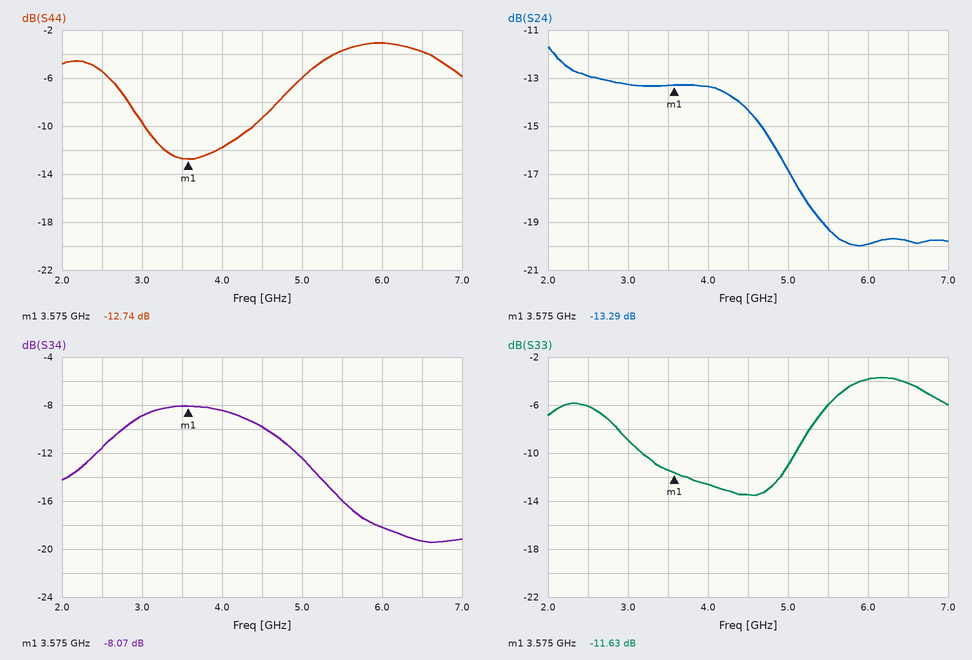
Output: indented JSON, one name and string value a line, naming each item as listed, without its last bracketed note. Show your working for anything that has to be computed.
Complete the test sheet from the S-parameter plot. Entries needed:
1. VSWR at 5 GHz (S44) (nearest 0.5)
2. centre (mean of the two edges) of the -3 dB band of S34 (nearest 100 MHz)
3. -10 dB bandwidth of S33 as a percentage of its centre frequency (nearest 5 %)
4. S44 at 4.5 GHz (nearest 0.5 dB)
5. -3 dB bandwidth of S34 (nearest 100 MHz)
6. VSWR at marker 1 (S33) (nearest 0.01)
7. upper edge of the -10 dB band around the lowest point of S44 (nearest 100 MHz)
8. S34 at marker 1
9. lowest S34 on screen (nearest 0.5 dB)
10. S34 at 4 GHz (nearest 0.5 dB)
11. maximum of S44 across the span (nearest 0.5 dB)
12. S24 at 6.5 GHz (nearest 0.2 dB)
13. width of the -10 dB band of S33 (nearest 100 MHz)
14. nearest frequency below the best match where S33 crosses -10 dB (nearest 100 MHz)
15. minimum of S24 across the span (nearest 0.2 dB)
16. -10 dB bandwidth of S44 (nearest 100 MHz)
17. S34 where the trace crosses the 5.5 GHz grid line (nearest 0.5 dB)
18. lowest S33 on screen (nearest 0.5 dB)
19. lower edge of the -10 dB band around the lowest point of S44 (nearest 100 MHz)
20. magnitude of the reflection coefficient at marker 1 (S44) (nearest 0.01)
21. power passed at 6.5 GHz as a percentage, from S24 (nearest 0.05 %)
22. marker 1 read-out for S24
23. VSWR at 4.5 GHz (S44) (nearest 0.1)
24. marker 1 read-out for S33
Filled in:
{
  "VSWR at 5 GHz (S44)": "|Γ| = 10^(-6/20) = 0.5012; VSWR = (1 + 0.5012)/(1 − 0.5012) ≈ 3.0",
  "centre (mean of the two edges) of the -3 dB band of S34": "3.7 GHz",
  "-10 dB bandwidth of S33 as a percentage of its centre frequency": "1.9 GHz / 4.15 GHz ≈ 45.8 %, so 45 % to the nearest 5 %",
  "S44 at 4.5 GHz": "-9.5 dB",
  "-3 dB bandwidth of S34": "4.8 GHz − 2.6 GHz = 2.2 GHz",
  "VSWR at marker 1 (S33)": "(1 + 0.2621)/(1 − 0.2621) ≈ 1.71",
  "upper edge of the -10 dB band around the lowest point of S44": "4.4 GHz",
  "S34 at marker 1": "-8.07 dB",
  "lowest S34 on screen": "-19.5 dB",
  "S34 at 4 GHz": "-8.5 dB",
  "maximum of S44 across the span": "-3.0 dB",
  "S24 at 6.5 GHz": "-19.8 dB",
  "width of the -10 dB band of S33": "5.1 GHz − 3.2 GHz = 1.9 GHz",
  "nearest frequency below the best match where S33 crosses -10 dB": "3.2 GHz",
  "minimum of S24 across the span": "-20.0 dB",
  "-10 dB bandwidth of S44": "4.4 GHz − 3.0 GHz = 1.4 GHz",
  "S34 where the trace crosses the 5.5 GHz grid line": "-16.0 dB",
  "lowest S33 on screen": "-13.5 dB",
  "lower edge of the -10 dB band around the lowest point of S44": "3.0 GHz",
  "magnitude of the reflection coefficient at marker 1 (S44)": "10^(-12.74/20) ≈ 0.23",
  "power passed at 6.5 GHz as a percentage, from S24": "10^(-19.8/10) ≈ 1.05 %",
  "marker 1 read-out for S24": "-13.29 dB",
  "VSWR at 4.5 GHz (S44)": "|Γ| = 10^(-9.5/20) = 0.3350; VSWR = (1 + 0.3350)/(1 − 0.3350) ≈ 2.0",
  "marker 1 read-out for S33": "-11.63 dB"
}
